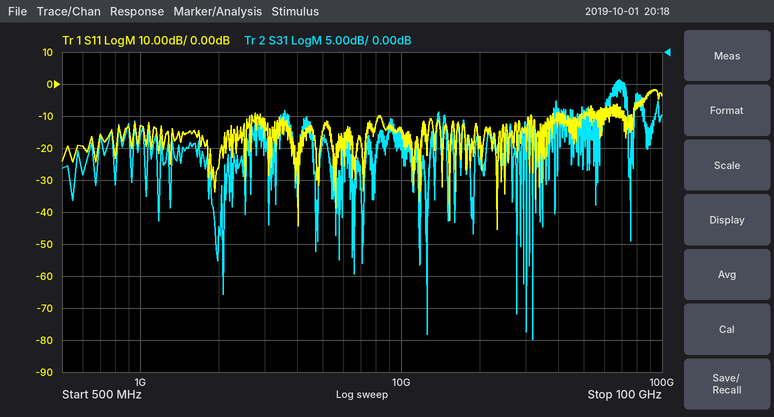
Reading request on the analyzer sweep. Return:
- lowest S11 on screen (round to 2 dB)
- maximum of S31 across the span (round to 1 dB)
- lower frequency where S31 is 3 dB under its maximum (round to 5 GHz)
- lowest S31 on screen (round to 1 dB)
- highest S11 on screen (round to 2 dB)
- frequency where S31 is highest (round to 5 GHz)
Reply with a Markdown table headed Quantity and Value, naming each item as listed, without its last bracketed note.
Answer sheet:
| Quantity | Value |
|---|---|
| lowest S11 on screen | -46 dB |
| maximum of S31 across the span | -4 dB |
| lower frequency where S31 is 3 dB under its maximum | 65 GHz |
| lowest S31 on screen | -45 dB |
| highest S11 on screen | -2 dB |
| frequency where S31 is highest | 70 GHz |
